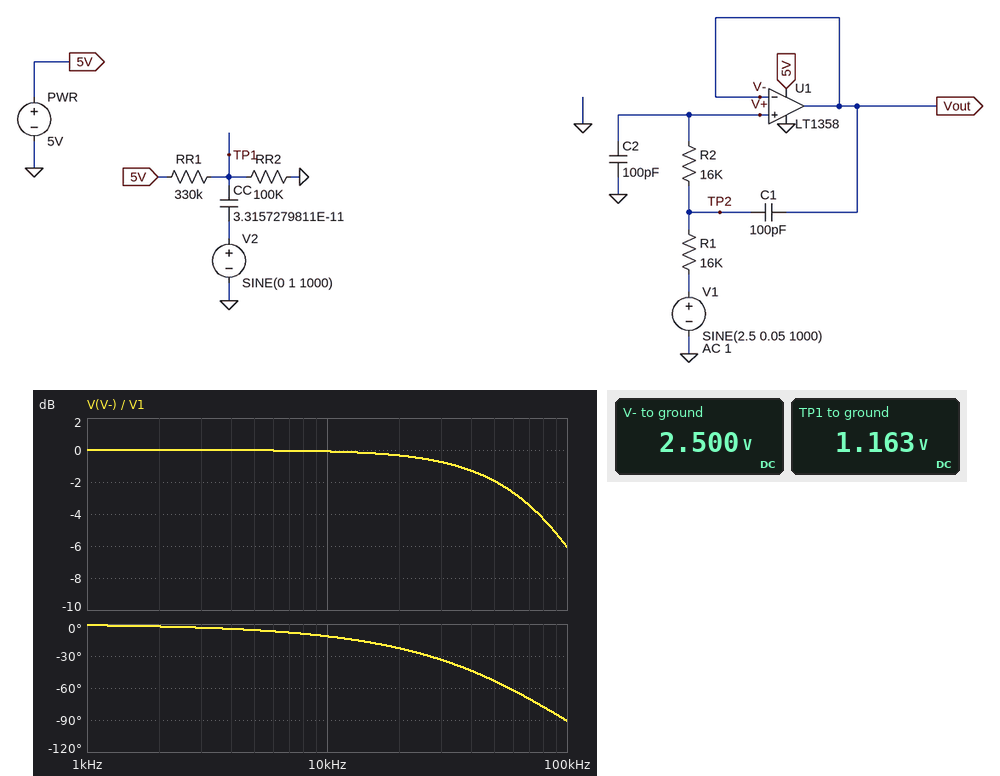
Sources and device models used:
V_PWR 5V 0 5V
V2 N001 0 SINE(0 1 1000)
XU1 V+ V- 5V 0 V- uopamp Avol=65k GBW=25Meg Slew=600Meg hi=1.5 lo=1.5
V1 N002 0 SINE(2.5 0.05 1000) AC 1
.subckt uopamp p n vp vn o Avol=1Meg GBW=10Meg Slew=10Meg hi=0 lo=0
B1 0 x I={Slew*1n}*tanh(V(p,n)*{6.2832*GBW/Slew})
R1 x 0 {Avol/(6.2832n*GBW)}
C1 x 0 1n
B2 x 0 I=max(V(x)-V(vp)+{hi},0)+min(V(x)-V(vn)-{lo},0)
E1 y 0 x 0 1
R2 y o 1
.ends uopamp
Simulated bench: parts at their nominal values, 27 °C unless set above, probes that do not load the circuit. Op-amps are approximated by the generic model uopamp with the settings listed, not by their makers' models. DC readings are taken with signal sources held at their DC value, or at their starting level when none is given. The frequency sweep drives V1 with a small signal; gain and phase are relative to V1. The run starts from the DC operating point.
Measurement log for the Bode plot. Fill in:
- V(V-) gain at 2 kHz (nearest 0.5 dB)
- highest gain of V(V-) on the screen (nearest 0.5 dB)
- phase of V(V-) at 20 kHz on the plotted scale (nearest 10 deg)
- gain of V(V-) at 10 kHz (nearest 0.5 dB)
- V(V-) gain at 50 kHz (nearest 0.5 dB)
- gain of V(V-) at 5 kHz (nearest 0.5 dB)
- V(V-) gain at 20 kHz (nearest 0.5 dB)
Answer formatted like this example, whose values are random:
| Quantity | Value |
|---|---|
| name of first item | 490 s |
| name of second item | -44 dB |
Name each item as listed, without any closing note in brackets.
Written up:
| Quantity | Value |
|---|---|
| V(V-) gain at 2 kHz | 0 dB |
| highest gain of V(V-) on the screen | 0 dB |
| phase of V(V-) at 20 kHz on the plotted scale | -20 deg |
| gain of V(V-) at 10 kHz | 0 dB |
| V(V-) gain at 50 kHz | -2.0 dB |
| gain of V(V-) at 5 kHz | 0 dB |
| V(V-) gain at 20 kHz | -0.5 dB |
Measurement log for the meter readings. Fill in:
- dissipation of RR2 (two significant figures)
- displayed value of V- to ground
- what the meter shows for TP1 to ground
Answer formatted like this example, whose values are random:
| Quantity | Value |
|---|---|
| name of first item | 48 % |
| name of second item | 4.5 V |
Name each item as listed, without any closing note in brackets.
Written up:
| Quantity | Value |
|---|---|
| dissipation of RR2 | 14 µW |
| displayed value of V- to ground | 2.500 V |
| what the meter shows for TP1 to ground | 1.163 V |
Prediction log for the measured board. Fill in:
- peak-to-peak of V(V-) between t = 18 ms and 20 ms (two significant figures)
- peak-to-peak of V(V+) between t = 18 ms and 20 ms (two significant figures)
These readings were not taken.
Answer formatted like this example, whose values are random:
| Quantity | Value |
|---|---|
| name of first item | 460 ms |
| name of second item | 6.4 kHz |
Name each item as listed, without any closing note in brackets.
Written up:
| Quantity | Value |
|---|---|
| peak-to-peak of V(V-) between t = 18 ms and 20 ms | 100 mV |
| peak-to-peak of V(V+) between t = 18 ms and 20 ms | 100 mV |
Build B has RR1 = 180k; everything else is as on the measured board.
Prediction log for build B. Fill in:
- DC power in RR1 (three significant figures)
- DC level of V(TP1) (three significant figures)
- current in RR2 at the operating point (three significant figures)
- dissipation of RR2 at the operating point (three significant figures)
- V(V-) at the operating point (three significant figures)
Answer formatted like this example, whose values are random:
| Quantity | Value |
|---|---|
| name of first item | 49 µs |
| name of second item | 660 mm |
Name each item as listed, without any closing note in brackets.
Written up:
| Quantity | Value |
|---|---|
| DC power in RR1 | 57.4 µW |
| DC level of V(TP1) | 1.79 V |
| current in RR2 at the operating point | 17.9 µA |
| dissipation of RR2 at the operating point | 31.9 µW |
| V(V-) at the operating point | 2.50 V |
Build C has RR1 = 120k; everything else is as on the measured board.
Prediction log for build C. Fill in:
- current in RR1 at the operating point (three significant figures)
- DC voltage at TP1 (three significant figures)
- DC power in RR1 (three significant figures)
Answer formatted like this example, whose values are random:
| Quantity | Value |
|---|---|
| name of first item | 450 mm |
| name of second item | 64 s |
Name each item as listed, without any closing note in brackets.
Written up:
| Quantity | Value |
|---|---|
| current in RR1 at the operating point | 22.7 µA |
| DC voltage at TP1 | 2.27 V |
| DC power in RR1 | 62.0 µW |
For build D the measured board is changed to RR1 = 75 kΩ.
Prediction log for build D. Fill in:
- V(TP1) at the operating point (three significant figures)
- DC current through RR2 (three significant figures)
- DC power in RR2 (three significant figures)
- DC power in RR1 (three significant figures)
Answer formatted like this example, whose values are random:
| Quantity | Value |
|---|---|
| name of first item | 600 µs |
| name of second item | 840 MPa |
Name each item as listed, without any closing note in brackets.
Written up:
| Quantity | Value |
|---|---|
| V(TP1) at the operating point | 2.86 V |
| DC current through RR2 | 28.6 µA |
| DC power in RR2 | 81.6 µW |
| DC power in RR1 | 61.2 µW |
